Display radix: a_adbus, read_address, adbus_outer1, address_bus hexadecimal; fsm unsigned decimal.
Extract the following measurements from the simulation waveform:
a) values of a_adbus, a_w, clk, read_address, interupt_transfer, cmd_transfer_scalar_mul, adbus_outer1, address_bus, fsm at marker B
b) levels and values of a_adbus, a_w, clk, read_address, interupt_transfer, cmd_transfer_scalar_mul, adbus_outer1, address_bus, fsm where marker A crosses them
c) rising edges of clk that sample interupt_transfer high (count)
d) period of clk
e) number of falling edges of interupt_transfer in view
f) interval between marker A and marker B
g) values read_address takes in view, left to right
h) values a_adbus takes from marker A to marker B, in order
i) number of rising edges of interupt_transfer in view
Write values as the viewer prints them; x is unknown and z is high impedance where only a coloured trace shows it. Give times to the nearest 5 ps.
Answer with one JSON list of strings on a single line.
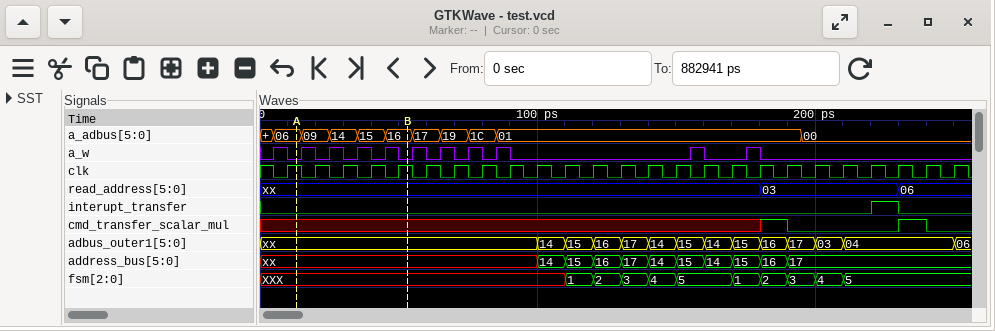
["a_adbus=16, a_w=0, clk=1, read_address=xx, interupt_transfer=0, cmd_transfer_scalar_mul=x, adbus_outer1=xx, address_bus=xx, fsm=XXX", "a_adbus=06, a_w=0, clk=1, read_address=xx, interupt_transfer=0, cmd_transfer_scalar_mul=x, adbus_outer1=xx, address_bus=xx, fsm=XXX", "1", "10 ps", "1", "40 ps", "xx, 03, 06", "06, 09, 14, 15, 16", "1"]
